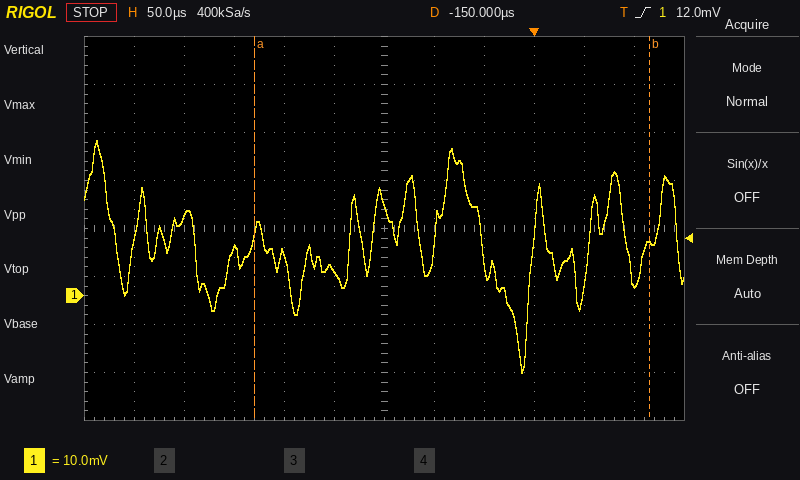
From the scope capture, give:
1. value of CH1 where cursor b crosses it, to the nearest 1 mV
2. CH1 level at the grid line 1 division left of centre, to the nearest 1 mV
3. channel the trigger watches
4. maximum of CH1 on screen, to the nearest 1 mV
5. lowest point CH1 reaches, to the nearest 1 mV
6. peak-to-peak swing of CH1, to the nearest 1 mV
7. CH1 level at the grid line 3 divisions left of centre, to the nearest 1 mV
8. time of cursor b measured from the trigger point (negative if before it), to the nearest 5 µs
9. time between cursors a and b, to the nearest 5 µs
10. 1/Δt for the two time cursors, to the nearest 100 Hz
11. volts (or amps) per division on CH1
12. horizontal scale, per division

11 mV
5 mV
CH1
32 mV
-16 mV
48 mV
10 mV
+115 µs
395 µs
2.5 kHz
10 mV
50 µs
